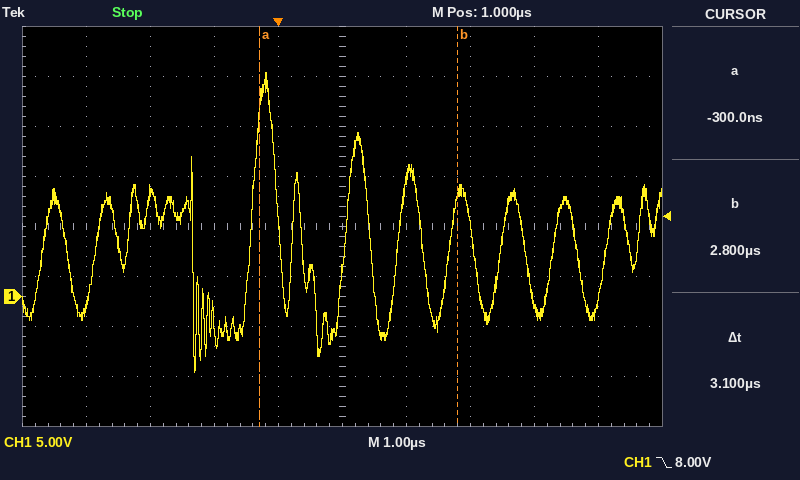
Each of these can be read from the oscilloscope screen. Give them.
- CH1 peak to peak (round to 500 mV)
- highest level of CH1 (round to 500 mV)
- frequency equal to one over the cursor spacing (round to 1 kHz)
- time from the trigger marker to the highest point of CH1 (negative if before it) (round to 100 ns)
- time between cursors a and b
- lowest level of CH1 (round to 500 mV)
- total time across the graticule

30.0 V
22.5 V
323 kHz
-200 ns
3.1 µs
-7.5 V
10 µs
